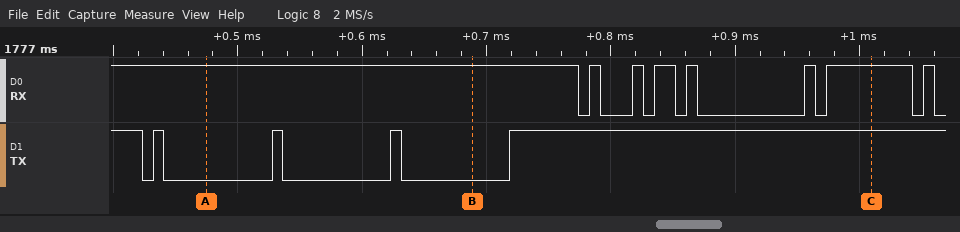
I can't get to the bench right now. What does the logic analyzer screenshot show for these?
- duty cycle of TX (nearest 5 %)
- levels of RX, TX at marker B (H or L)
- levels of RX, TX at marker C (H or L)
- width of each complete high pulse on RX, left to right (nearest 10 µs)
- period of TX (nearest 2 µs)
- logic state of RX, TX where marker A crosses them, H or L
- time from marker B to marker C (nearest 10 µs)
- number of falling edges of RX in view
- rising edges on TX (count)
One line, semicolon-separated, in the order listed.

10 %; RX=H, TX=L; RX=H, TX=H; 10 µs, 10 µs, 20 µs, 10 µs, 10 µs, 70 µs, 10 µs; 96 µs; RX=H, TX=L; 320 µs; 8; 4
